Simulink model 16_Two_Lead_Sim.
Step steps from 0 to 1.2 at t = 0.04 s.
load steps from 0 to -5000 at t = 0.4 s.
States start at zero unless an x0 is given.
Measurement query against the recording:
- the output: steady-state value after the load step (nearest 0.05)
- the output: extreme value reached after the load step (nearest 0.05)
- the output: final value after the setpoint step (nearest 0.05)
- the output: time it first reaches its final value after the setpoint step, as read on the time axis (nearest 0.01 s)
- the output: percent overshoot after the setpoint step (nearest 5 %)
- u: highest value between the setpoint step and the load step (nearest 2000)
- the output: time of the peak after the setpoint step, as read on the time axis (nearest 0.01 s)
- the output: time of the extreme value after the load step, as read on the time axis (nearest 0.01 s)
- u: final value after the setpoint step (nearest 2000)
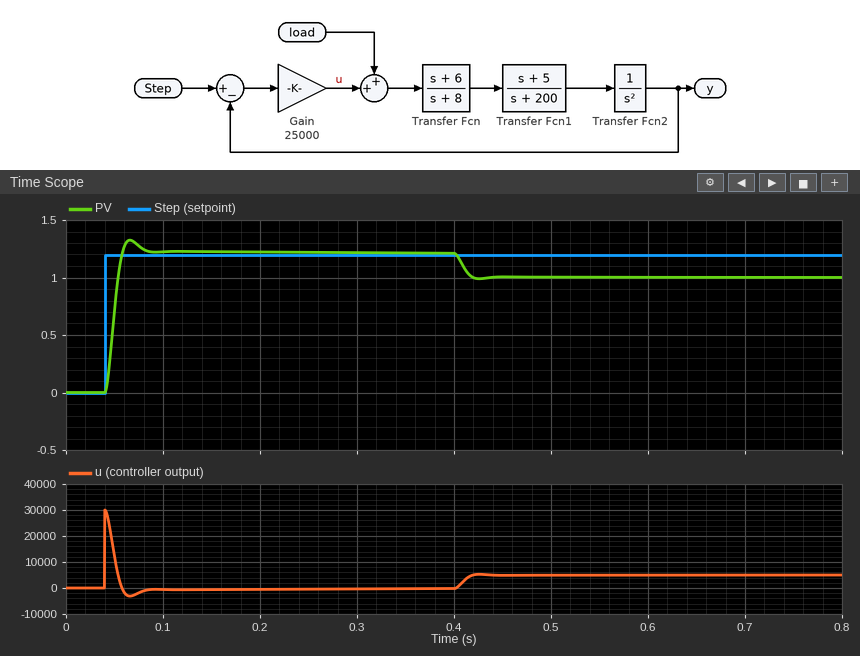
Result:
1.00
1.00
1.20
0.06 s
10 %
30000
0.07 s
0.43 s
0
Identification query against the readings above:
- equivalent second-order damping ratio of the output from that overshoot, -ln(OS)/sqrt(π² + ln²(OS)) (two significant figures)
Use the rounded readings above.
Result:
0.59
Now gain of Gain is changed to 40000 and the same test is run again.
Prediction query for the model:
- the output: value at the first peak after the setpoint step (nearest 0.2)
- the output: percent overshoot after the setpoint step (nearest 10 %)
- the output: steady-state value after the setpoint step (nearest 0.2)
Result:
1.4
20 %
1.2
